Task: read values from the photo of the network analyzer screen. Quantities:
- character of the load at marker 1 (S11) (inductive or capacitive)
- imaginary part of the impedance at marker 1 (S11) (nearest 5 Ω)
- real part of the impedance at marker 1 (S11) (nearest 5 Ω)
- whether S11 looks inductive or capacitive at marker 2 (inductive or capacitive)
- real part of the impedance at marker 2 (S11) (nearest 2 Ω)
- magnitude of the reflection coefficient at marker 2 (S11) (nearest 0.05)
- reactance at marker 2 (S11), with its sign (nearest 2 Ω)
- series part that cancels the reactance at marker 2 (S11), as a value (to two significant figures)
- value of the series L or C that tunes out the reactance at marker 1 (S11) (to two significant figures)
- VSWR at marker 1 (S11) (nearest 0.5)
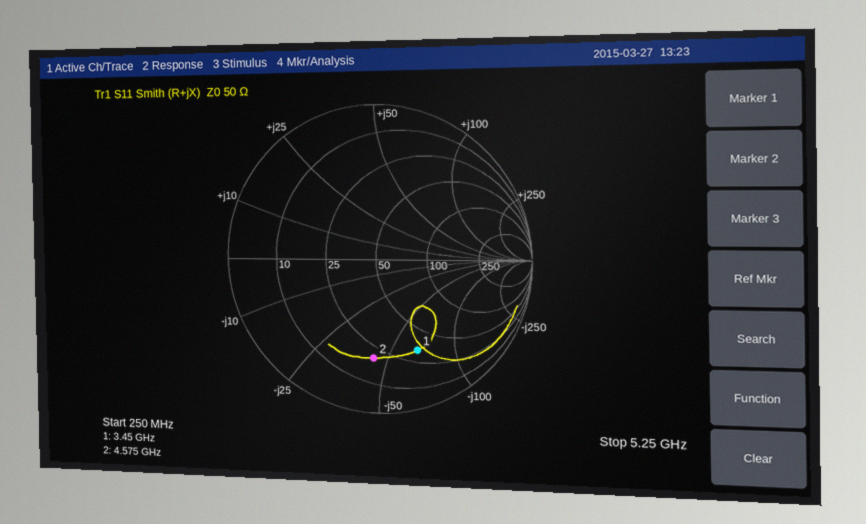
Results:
capacitive
-65 Ω
35 Ω
capacitive
20 Ω
0.65
-44 Ω
1.5 nH
3.0 nH
4.5
